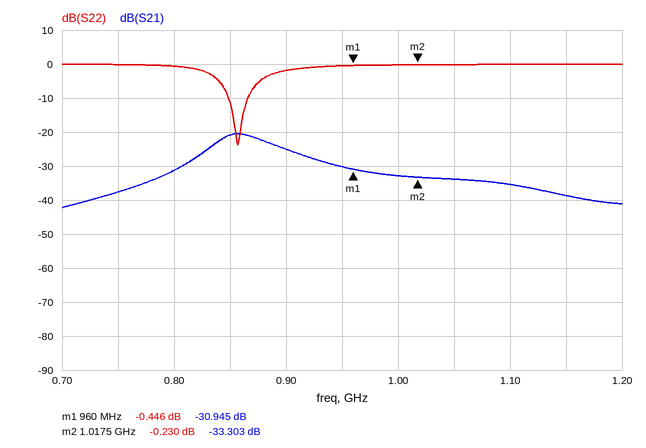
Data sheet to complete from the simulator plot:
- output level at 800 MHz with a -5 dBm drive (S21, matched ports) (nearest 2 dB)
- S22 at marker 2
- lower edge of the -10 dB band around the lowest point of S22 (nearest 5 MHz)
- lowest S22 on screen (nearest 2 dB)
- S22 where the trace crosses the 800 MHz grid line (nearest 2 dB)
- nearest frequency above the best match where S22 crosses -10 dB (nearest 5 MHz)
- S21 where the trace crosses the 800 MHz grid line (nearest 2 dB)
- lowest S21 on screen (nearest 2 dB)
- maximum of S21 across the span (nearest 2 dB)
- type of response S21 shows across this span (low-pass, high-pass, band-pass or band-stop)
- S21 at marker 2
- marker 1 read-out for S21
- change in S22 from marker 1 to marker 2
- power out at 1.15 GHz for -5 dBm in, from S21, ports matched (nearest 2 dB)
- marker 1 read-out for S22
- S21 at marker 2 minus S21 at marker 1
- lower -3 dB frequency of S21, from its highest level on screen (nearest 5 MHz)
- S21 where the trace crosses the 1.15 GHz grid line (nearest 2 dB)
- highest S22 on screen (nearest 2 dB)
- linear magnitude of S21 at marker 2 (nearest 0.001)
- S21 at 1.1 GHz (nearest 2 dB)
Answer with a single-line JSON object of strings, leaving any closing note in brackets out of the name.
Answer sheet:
{"output level at 800 MHz with a -5 dBm drive (S21, matched ports)": "-36 dBm", "S22 at marker 2": "-0.230 dB", "lower edge of the -10 dB band around the lowest point of S22": "850 MHz", "lowest S22 on screen": "-24 dB", "S22 where the trace crosses the 800 MHz grid line": "0 dB", "nearest frequency above the best match where S22 crosses -10 dB": "865 MHz", "S21 where the trace crosses the 800 MHz grid line": "-32 dB", "lowest S21 on screen": "-42 dB", "maximum of S21 across the span": "-20 dB", "type of response S21 shows across this span": "band-pass", "S21 at marker 2": "-33.303 dB", "marker 1 read-out for S21": "-30.945 dB", "change in S22 from marker 1 to marker 2": "0.216 dB", "power out at 1.15 GHz for -5 dBm in, from S21, ports matched": "-44 dBm", "marker 1 read-out for S22": "-0.446 dB", "S21 at marker 2 minus S21 at marker 1": "-2.358 dB", "lower -3 dB frequency of S21, from its highest level on screen": "835 MHz", "S21 where the trace crosses the 1.15 GHz grid line": "-38 dB", "highest S22 on screen": "0 dB", "linear magnitude of S21 at marker 2": "0.022", "S21 at 1.1 GHz": "-36 dB"}
